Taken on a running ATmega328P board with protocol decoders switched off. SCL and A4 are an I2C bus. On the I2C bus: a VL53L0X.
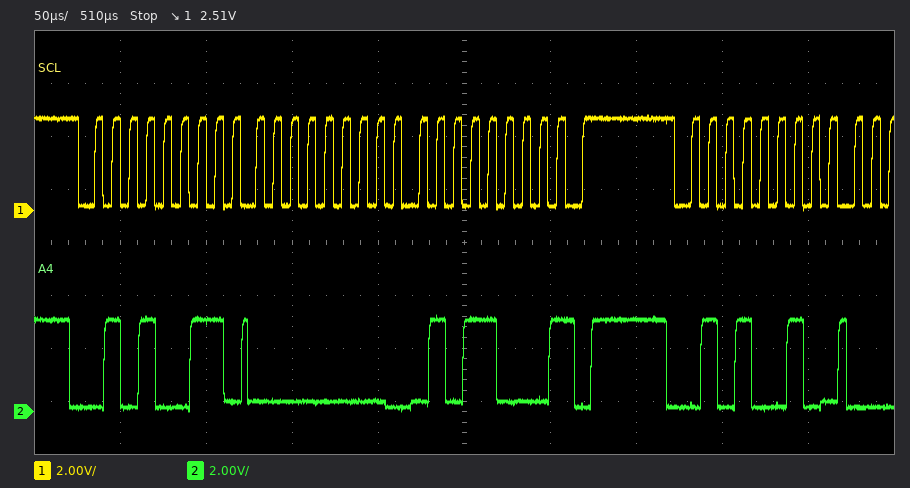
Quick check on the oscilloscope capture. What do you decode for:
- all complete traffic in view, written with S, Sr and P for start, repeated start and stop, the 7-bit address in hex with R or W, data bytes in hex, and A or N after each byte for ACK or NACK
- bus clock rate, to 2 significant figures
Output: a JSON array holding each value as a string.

["S 29R A 00 A 58 N P S 29W A", "100 kHz"]
